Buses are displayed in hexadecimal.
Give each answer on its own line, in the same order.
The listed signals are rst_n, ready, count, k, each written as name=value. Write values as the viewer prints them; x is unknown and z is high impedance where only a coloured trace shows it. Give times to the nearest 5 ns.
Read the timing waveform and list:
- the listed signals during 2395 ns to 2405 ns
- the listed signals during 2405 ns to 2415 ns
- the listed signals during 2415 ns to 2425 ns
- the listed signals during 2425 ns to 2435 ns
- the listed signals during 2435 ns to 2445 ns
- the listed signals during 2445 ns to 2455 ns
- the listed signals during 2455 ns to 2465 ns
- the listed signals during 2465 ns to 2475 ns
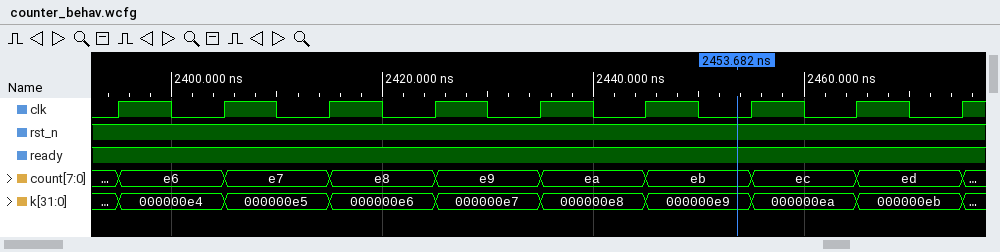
rst_n=1, ready=1, count=e6, k=000000e4
rst_n=1, ready=1, count=e7, k=000000e5
rst_n=1, ready=1, count=e8, k=000000e6
rst_n=1, ready=1, count=e9, k=000000e7
rst_n=1, ready=1, count=ea, k=000000e8
rst_n=1, ready=1, count=eb, k=000000e9
rst_n=1, ready=1, count=ec, k=000000ea
rst_n=1, ready=1, count=ed, k=000000eb
